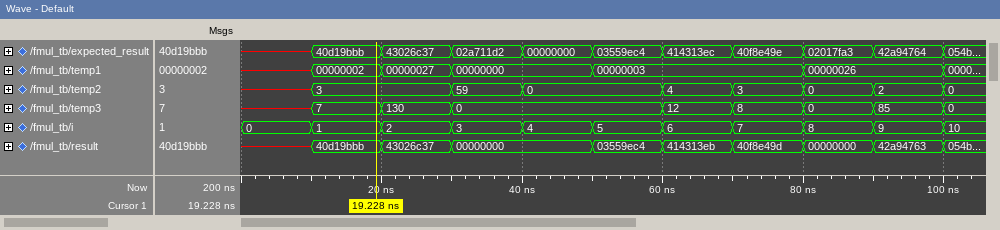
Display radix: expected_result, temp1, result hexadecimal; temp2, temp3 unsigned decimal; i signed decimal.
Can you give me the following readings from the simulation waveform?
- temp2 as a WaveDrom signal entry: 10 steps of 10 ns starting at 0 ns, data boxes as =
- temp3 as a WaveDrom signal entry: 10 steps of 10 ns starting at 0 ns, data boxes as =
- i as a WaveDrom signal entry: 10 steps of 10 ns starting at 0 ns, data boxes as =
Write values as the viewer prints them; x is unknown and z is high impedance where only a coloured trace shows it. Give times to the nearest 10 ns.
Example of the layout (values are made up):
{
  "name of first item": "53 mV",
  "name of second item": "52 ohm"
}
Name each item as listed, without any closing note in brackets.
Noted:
{
  "temp2 as a WaveDrom signal entry: 10 steps of 10 ns starting at 0 ns, data boxes as =": "{name: 'temp2', wave: 'x=.==.====', data: '3 59 0 4 3 0 2'}",
  "temp3 as a WaveDrom signal entry: 10 steps of 10 ns starting at 0 ns, data boxes as =": "{name: 'temp3', wave: 'x===..====', data: '7 130 0 12 8 0 85'}",
  "i as a WaveDrom signal entry: 10 steps of 10 ns starting at 0 ns, data boxes as =": "{name: 'i', wave: '==========', data: '0 1 2 3 4 5 6 7 8 9'}"
}
